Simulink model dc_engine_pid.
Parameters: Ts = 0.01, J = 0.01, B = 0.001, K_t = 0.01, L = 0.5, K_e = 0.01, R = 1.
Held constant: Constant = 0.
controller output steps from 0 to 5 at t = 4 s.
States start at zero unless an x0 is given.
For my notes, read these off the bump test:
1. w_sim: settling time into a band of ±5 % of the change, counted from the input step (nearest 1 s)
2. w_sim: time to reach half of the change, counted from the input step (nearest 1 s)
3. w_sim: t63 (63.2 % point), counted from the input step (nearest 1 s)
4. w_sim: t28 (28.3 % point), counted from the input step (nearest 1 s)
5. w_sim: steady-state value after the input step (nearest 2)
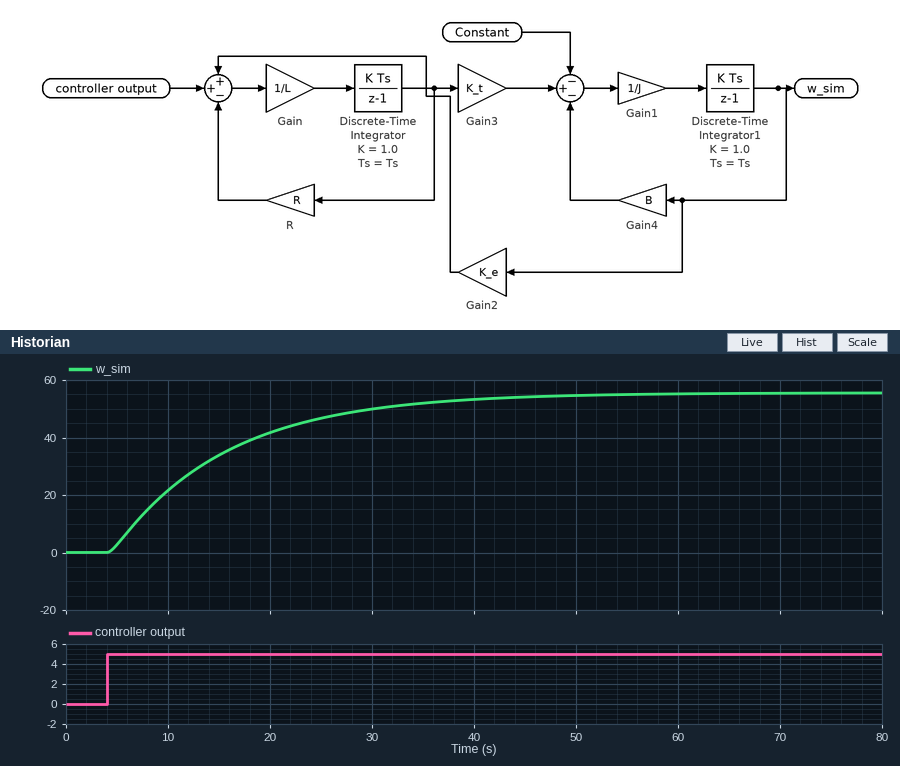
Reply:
34 s
8 s
12 s
4 s
56
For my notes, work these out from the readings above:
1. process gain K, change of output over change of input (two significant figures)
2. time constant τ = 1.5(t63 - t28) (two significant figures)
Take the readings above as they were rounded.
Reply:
11
12 s
